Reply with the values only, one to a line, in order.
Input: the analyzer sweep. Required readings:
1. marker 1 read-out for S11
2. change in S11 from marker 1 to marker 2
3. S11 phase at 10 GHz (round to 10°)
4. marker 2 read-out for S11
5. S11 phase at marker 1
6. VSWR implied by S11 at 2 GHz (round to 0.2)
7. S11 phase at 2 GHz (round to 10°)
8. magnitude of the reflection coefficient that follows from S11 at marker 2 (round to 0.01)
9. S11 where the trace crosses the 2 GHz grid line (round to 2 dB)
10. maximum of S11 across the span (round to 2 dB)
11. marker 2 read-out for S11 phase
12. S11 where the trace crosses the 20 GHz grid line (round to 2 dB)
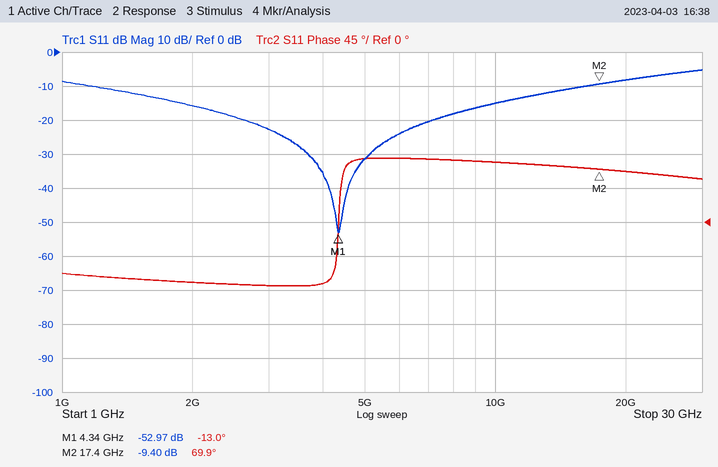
-52.97 dB
43.57 dB
80°
-9.40 dB
-13.0°
1.4
-80°
0.34
-16 dB
-6 dB
69.9°
-8 dB
